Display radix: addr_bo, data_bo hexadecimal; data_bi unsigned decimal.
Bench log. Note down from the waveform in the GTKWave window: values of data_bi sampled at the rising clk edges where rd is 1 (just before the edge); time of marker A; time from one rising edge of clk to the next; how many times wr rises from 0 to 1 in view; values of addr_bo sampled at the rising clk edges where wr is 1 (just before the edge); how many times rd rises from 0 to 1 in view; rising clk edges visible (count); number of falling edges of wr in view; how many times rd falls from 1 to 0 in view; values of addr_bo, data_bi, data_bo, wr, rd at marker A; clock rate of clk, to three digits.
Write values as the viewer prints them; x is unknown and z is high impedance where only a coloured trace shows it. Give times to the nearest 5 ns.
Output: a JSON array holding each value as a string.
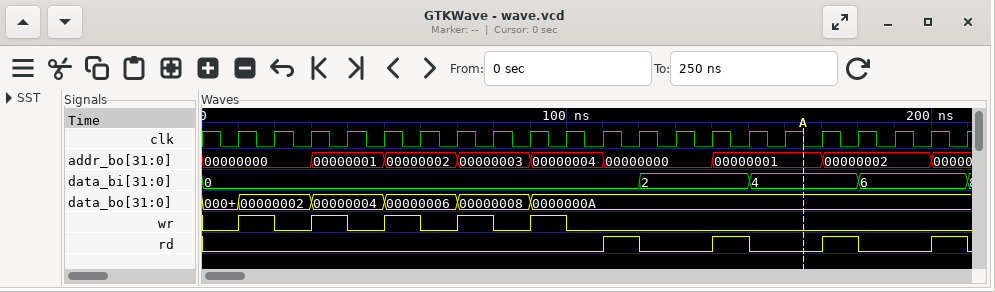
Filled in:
["0, 2, 4, 6", "165 ns", "10 ns", "5", "00000000, 00000001, 00000002, 00000003, 00000004", "4", "21", "5", "4", "addr_bo=00000001, data_bi=4, data_bo=0000000A, wr=0, rd=0", "100 MHz"]
